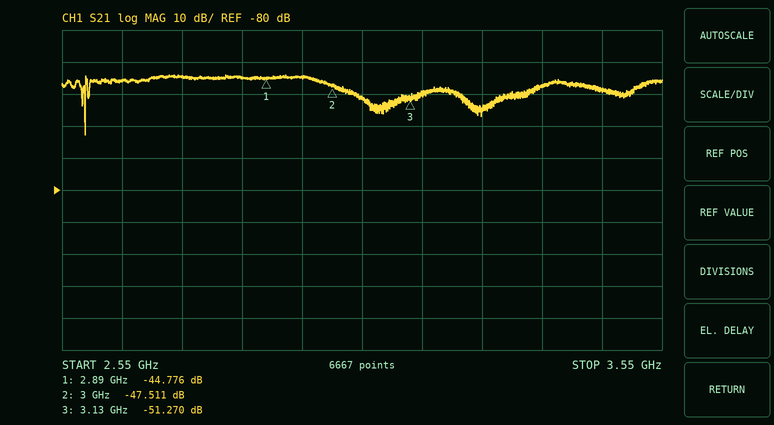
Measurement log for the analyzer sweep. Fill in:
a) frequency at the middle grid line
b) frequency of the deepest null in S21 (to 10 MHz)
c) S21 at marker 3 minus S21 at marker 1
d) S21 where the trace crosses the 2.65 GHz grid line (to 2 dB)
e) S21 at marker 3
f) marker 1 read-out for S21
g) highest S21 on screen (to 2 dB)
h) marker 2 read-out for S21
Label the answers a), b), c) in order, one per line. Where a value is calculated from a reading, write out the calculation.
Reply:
a) 3.05 GHz
b) 2.59 GHz
c) -51.27 − (-44.776) = -6.494 dB
d) -46 dB
e) -51.270 dB
f) -44.776 dB
g) -44 dB
h) -47.511 dB
